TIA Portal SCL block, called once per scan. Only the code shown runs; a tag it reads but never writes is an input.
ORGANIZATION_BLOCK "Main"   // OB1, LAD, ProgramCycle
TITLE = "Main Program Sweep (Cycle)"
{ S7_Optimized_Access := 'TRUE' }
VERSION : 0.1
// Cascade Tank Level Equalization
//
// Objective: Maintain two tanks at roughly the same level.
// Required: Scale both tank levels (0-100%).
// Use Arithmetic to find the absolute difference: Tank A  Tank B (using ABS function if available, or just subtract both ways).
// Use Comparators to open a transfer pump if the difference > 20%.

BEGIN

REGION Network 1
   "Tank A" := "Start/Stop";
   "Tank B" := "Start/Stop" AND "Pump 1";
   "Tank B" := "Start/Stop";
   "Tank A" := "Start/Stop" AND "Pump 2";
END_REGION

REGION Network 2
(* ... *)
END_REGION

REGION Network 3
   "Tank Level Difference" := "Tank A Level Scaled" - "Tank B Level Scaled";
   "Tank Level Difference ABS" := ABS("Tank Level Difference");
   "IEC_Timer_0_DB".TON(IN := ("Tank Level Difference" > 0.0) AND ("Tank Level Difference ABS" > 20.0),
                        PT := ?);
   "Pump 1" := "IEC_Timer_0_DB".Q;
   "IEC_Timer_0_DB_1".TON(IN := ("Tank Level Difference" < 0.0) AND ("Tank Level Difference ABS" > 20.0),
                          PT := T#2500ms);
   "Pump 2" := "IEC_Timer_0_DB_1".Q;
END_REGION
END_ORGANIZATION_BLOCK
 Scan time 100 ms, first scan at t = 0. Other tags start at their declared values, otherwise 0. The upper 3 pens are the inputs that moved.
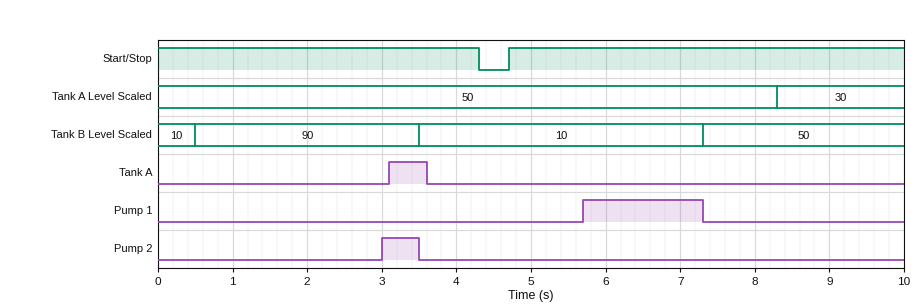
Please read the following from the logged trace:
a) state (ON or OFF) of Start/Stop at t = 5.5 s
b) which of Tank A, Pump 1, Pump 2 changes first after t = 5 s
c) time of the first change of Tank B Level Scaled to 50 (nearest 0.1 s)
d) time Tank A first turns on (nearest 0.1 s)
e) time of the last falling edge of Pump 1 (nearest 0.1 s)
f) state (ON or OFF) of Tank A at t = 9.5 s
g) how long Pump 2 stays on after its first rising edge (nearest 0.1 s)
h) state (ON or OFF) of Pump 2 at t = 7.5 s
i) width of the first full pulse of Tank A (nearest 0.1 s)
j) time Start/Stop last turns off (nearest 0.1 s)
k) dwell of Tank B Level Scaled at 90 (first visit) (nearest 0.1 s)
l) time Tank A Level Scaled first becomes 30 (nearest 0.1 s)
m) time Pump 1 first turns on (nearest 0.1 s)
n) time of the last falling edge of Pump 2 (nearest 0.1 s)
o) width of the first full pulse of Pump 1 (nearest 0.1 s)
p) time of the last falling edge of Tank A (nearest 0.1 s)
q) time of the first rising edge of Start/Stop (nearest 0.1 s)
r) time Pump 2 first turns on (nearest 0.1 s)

ON
Pump 1
7.3 s
3.1 s
7.3 s
OFF
0.5 s
OFF
0.5 s
4.3 s
3.0 s
8.3 s
5.7 s
3.5 s
1.6 s
3.6 s
4.7 s
3.0 s
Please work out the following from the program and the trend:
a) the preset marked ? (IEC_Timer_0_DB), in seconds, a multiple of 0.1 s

2.2 s
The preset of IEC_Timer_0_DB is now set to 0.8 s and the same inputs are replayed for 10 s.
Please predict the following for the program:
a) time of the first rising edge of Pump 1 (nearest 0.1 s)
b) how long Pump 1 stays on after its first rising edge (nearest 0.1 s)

4.3 s
3.0 s
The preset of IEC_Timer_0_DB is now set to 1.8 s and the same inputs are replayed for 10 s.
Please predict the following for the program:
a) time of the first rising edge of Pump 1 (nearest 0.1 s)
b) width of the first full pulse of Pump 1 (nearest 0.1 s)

5.3 s
2.0 s
